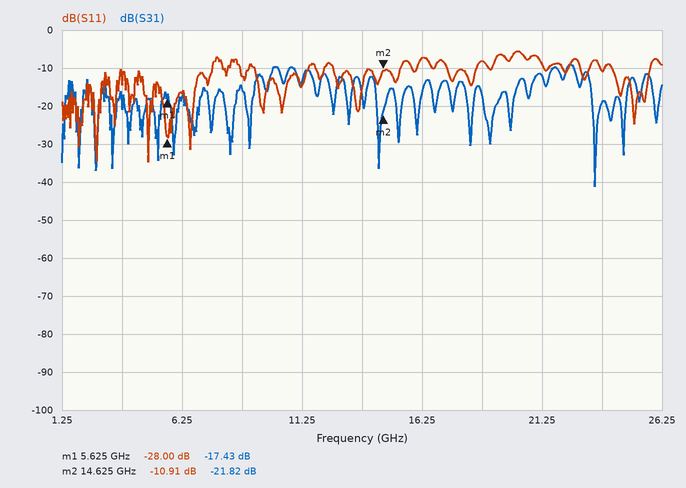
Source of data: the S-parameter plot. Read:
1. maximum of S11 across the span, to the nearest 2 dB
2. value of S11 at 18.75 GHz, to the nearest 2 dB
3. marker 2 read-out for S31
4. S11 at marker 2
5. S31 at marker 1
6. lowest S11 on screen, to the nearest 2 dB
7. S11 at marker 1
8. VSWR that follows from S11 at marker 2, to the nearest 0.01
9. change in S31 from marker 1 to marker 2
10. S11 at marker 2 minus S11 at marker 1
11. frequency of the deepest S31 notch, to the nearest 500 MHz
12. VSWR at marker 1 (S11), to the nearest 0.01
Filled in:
-6 dB
-8 dB
-21.82 dB
-10.91 dB
-17.43 dB
-34 dB
-28.00 dB
1.80
-4.39 dB
17.09 dB
23.5 GHz
1.08
